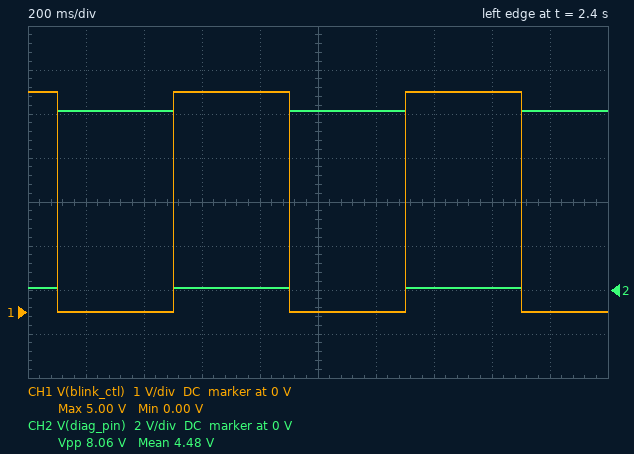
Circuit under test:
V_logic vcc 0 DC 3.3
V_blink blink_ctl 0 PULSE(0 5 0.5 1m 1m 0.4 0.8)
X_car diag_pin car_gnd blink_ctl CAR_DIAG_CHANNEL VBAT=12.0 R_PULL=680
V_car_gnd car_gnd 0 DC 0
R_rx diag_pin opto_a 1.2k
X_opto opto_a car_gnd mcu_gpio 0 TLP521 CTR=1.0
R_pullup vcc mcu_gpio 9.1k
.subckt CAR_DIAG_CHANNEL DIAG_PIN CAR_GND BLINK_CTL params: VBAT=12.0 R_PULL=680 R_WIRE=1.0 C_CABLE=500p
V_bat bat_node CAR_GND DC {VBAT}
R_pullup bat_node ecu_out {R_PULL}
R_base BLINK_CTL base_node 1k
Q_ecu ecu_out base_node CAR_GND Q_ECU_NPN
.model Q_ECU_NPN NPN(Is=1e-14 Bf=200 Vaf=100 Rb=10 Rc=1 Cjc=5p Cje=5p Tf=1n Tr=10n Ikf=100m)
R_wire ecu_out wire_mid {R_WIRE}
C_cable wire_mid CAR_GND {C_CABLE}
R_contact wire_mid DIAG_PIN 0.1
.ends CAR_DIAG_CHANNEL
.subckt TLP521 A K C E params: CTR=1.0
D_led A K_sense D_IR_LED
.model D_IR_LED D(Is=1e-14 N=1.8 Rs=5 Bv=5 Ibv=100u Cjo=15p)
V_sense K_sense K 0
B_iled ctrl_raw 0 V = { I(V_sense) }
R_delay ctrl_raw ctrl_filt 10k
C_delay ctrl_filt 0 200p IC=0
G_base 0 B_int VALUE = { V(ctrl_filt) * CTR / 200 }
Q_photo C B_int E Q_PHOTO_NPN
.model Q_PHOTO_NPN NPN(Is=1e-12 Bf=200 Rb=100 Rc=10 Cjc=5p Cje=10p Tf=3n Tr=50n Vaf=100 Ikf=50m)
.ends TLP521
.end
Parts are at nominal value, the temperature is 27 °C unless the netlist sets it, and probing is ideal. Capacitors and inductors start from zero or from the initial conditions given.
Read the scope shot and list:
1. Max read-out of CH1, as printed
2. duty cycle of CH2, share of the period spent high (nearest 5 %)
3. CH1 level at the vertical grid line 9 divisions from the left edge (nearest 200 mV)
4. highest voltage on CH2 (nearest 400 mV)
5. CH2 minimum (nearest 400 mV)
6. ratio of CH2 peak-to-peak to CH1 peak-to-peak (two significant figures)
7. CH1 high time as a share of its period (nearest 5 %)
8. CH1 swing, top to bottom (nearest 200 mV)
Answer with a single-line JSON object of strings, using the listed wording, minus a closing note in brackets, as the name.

{"Max read-out of CH1, as printed": "5.00 V", "duty cycle of CH2, share of the period spent high": "50 %", "CH1 level at the vertical grid line 9 divisions from the left edge": "0 V", "highest voltage on CH2": "8.0 V", "CH2 minimum": "0 V", "ratio of CH2 peak-to-peak to CH1 peak-to-peak": "1.6", "CH1 high time as a share of its period": "50 %", "CH1 swing, top to bottom": "5.0 V"}
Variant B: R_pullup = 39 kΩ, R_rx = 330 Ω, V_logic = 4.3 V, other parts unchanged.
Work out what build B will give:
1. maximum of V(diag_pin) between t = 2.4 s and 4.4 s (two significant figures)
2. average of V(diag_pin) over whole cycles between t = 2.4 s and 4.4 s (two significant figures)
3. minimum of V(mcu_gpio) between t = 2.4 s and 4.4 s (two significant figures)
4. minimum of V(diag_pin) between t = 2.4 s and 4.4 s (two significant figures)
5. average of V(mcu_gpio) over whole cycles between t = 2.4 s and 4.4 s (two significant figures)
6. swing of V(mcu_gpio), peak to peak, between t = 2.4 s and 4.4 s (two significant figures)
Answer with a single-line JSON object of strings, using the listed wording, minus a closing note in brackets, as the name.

{"maximum of V(diag_pin) between t = 2.4 s and 4.4 s": "4.8 V", "average of V(diag_pin) over whole cycles between t = 2.4 s and 4.4 s": "2.4 V", "minimum of V(mcu_gpio) between t = 2.4 s and 4.4 s": "38 mV", "minimum of V(diag_pin) between t = 2.4 s and 4.4 s": "70 mV", "average of V(mcu_gpio) over whole cycles between t = 2.4 s and 4.4 s": "2.2 V", "swing of V(mcu_gpio), peak to peak, between t = 2.4 s and 4.4 s": "4.3 V"}
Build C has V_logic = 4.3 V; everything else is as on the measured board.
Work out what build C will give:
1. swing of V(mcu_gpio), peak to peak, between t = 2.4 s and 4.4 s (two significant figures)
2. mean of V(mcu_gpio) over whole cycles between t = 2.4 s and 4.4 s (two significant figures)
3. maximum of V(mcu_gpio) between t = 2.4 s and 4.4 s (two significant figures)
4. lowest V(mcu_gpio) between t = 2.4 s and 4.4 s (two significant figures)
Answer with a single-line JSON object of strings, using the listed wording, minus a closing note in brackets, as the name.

{"swing of V(mcu_gpio), peak to peak, between t = 2.4 s and 4.4 s": "4.2 V", "mean of V(mcu_gpio) over whole cycles between t = 2.4 s and 4.4 s": "2.2 V", "maximum of V(mcu_gpio) between t = 2.4 s and 4.4 s": "4.3 V", "lowest V(mcu_gpio) between t = 2.4 s and 4.4 s": "82 mV"}
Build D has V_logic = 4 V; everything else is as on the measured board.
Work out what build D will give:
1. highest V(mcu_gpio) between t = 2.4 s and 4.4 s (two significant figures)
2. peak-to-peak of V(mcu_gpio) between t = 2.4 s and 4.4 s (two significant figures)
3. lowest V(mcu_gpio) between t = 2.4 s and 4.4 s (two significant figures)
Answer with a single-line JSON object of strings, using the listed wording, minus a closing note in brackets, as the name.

{"highest V(mcu_gpio) between t = 2.4 s and 4.4 s": "4.0 V", "peak-to-peak of V(mcu_gpio) between t = 2.4 s and 4.4 s": "3.9 V", "lowest V(mcu_gpio) between t = 2.4 s and 4.4 s": "80 mV"}
